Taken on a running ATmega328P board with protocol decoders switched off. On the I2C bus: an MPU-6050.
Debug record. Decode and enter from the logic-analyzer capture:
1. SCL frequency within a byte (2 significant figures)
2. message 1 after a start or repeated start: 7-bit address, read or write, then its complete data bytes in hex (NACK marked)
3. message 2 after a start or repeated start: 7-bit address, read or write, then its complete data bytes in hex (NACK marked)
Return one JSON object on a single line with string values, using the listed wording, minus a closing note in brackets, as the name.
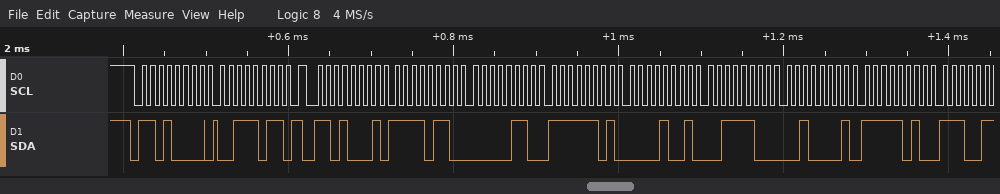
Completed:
{"SCL frequency within a byte": "100 kHz", "message 1 after a start or repeated start: 7-bit address, read or write, then its complete data bytes in hex": "0x68 write: 3B", "message 2 after a start or repeated start: 7-bit address, read or write, then its complete data bytes in hex": "0x68 read: F6 06 FD 09 3C 21 FA"}
